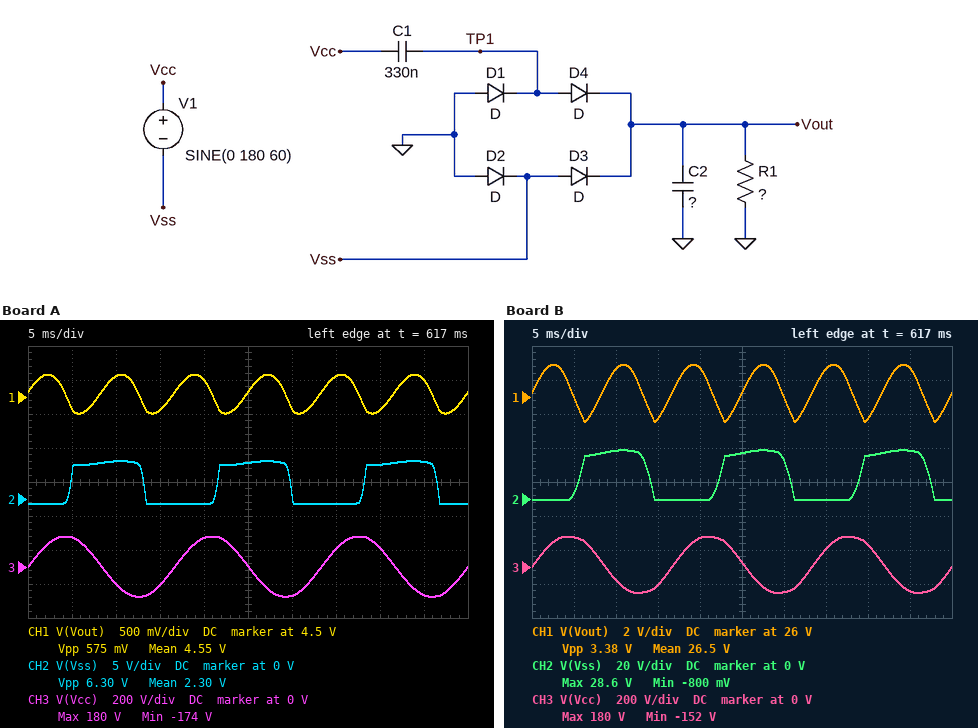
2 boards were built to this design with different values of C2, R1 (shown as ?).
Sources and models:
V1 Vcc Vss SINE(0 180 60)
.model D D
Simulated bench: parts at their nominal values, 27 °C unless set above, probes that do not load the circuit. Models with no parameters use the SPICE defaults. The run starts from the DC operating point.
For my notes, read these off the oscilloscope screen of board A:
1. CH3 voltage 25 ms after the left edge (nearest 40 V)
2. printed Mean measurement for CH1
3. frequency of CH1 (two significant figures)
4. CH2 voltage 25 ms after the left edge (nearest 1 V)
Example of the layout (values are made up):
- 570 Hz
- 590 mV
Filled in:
- 0 V
- 4.55 V
- 120 Hz
- 5 V
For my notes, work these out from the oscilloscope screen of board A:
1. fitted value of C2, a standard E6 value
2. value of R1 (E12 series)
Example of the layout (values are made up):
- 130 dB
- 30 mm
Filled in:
- 47 µF
- 330 Ω
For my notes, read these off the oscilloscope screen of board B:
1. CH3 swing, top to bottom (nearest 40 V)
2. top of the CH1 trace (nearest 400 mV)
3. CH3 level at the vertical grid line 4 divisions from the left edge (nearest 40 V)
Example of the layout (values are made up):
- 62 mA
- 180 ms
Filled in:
- 320 V
- 28.0 V
- 160 V
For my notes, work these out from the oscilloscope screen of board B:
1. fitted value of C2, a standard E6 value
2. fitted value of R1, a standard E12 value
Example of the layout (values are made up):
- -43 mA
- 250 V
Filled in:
- 10 µF
- 2.2 kΩ
